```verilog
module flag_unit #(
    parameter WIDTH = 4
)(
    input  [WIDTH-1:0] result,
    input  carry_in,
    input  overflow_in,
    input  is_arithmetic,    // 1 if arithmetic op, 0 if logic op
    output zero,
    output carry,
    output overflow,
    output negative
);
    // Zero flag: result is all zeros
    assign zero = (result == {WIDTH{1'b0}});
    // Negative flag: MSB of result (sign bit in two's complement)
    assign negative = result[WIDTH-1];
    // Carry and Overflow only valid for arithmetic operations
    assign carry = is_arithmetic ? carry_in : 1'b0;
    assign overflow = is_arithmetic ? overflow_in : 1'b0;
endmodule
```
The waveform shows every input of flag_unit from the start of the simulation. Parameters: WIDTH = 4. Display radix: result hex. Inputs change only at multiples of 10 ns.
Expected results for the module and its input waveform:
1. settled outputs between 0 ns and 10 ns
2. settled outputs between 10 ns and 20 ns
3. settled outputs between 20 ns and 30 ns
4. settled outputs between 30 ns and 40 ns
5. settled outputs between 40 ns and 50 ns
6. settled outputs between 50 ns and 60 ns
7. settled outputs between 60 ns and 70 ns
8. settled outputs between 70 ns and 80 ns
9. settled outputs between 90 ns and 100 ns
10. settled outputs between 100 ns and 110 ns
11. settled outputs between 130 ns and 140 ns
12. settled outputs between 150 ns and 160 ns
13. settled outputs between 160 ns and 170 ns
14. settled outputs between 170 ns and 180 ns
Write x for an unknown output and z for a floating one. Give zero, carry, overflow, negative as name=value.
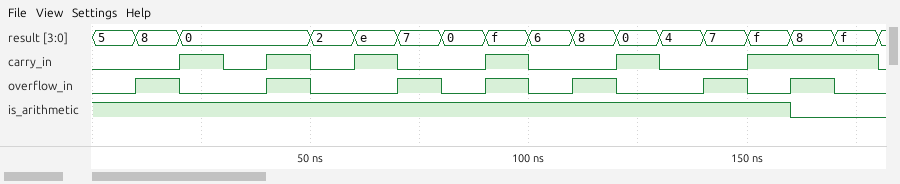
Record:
zero=0, carry=0, overflow=0, negative=0
zero=0, carry=0, overflow=1, negative=1
zero=1, carry=1, overflow=0, negative=0
zero=1, carry=0, overflow=0, negative=0
zero=1, carry=1, overflow=1, negative=0
zero=0, carry=0, overflow=0, negative=0
zero=0, carry=1, overflow=0, negative=1
zero=0, carry=0, overflow=1, negative=0
zero=0, carry=1, overflow=1, negative=1
zero=0, carry=0, overflow=0, negative=0
zero=0, carry=0, overflow=0, negative=0
zero=0, carry=1, overflow=0, negative=1
zero=0, carry=0, overflow=0, negative=1
zero=0, carry=0, overflow=0, negative=1
